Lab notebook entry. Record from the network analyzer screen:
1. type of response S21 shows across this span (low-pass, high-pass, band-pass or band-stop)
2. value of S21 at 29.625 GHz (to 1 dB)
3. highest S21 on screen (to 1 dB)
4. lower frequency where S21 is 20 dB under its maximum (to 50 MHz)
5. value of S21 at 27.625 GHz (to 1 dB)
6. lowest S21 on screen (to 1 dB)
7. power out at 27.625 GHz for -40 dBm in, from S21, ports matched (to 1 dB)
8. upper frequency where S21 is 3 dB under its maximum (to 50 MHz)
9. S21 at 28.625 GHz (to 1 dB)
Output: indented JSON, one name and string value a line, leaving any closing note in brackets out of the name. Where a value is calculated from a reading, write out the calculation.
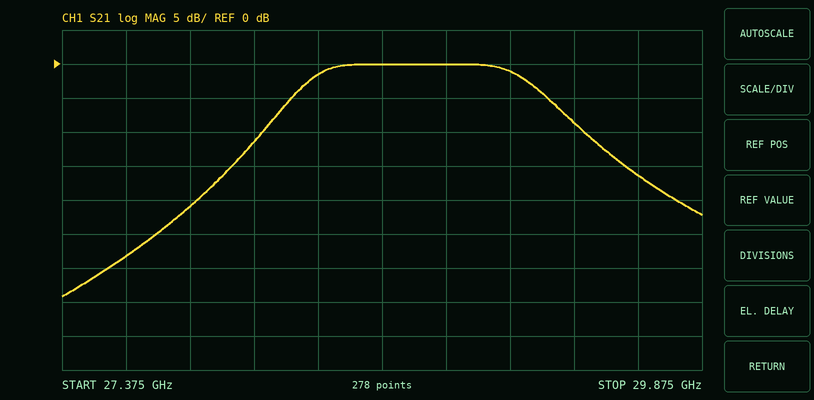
{
  "type of response S21 shows across this span": "band-pass",
  "value of S21 at 29.625 GHz": "-16 dB",
  "highest S21 on screen": "0 dB",
  "lower frequency where S21 is 20 dB under its maximum": "27.90 GHz",
  "value of S21 at 27.625 GHz": "-28 dB",
  "lowest S21 on screen": "-34 dB",
  "power out at 27.625 GHz for -40 dBm in, from S21, ports matched": "-40 dBm + (-28 dB) = -68 dBm",
  "upper frequency where S21 is 3 dB under its maximum": "29.20 GHz",
  "S21 at 28.625 GHz": "0 dB"
}
